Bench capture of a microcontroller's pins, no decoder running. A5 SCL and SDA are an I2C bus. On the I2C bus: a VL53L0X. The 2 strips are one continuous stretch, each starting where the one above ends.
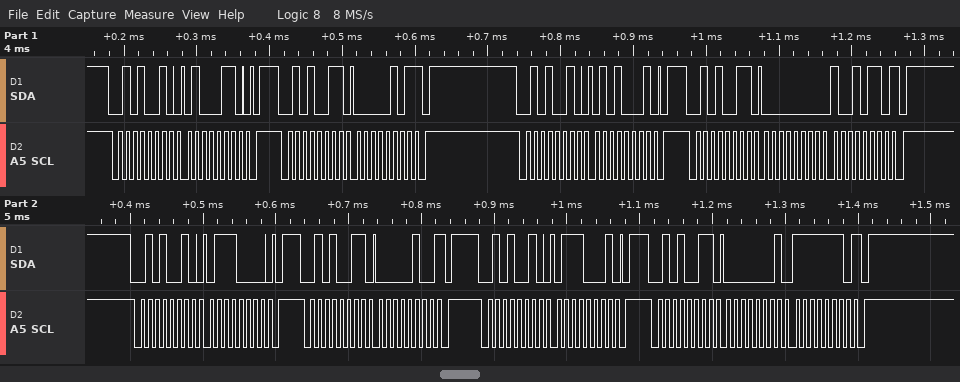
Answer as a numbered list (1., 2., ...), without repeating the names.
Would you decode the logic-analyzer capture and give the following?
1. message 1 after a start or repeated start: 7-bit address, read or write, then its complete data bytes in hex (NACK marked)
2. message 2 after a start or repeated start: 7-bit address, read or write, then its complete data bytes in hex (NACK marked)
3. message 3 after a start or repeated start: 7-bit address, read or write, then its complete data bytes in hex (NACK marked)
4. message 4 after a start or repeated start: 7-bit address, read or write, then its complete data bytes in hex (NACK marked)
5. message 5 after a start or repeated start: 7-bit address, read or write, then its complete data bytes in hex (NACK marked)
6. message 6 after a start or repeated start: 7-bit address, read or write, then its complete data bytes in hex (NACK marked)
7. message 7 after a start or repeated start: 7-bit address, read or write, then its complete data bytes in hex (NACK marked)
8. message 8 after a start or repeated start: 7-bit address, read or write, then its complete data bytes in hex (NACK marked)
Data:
1. 0x29 write: 46
2. 0x29 read: 05 NACK
3. 0x29 write: 51
4. 0x29 read: 00 96 NACK
5. 0x29 write: 70
6. 0x29 read: 04 NACK
7. 0x29 write: 71
8. 0x29 read: 01 FE NACK
